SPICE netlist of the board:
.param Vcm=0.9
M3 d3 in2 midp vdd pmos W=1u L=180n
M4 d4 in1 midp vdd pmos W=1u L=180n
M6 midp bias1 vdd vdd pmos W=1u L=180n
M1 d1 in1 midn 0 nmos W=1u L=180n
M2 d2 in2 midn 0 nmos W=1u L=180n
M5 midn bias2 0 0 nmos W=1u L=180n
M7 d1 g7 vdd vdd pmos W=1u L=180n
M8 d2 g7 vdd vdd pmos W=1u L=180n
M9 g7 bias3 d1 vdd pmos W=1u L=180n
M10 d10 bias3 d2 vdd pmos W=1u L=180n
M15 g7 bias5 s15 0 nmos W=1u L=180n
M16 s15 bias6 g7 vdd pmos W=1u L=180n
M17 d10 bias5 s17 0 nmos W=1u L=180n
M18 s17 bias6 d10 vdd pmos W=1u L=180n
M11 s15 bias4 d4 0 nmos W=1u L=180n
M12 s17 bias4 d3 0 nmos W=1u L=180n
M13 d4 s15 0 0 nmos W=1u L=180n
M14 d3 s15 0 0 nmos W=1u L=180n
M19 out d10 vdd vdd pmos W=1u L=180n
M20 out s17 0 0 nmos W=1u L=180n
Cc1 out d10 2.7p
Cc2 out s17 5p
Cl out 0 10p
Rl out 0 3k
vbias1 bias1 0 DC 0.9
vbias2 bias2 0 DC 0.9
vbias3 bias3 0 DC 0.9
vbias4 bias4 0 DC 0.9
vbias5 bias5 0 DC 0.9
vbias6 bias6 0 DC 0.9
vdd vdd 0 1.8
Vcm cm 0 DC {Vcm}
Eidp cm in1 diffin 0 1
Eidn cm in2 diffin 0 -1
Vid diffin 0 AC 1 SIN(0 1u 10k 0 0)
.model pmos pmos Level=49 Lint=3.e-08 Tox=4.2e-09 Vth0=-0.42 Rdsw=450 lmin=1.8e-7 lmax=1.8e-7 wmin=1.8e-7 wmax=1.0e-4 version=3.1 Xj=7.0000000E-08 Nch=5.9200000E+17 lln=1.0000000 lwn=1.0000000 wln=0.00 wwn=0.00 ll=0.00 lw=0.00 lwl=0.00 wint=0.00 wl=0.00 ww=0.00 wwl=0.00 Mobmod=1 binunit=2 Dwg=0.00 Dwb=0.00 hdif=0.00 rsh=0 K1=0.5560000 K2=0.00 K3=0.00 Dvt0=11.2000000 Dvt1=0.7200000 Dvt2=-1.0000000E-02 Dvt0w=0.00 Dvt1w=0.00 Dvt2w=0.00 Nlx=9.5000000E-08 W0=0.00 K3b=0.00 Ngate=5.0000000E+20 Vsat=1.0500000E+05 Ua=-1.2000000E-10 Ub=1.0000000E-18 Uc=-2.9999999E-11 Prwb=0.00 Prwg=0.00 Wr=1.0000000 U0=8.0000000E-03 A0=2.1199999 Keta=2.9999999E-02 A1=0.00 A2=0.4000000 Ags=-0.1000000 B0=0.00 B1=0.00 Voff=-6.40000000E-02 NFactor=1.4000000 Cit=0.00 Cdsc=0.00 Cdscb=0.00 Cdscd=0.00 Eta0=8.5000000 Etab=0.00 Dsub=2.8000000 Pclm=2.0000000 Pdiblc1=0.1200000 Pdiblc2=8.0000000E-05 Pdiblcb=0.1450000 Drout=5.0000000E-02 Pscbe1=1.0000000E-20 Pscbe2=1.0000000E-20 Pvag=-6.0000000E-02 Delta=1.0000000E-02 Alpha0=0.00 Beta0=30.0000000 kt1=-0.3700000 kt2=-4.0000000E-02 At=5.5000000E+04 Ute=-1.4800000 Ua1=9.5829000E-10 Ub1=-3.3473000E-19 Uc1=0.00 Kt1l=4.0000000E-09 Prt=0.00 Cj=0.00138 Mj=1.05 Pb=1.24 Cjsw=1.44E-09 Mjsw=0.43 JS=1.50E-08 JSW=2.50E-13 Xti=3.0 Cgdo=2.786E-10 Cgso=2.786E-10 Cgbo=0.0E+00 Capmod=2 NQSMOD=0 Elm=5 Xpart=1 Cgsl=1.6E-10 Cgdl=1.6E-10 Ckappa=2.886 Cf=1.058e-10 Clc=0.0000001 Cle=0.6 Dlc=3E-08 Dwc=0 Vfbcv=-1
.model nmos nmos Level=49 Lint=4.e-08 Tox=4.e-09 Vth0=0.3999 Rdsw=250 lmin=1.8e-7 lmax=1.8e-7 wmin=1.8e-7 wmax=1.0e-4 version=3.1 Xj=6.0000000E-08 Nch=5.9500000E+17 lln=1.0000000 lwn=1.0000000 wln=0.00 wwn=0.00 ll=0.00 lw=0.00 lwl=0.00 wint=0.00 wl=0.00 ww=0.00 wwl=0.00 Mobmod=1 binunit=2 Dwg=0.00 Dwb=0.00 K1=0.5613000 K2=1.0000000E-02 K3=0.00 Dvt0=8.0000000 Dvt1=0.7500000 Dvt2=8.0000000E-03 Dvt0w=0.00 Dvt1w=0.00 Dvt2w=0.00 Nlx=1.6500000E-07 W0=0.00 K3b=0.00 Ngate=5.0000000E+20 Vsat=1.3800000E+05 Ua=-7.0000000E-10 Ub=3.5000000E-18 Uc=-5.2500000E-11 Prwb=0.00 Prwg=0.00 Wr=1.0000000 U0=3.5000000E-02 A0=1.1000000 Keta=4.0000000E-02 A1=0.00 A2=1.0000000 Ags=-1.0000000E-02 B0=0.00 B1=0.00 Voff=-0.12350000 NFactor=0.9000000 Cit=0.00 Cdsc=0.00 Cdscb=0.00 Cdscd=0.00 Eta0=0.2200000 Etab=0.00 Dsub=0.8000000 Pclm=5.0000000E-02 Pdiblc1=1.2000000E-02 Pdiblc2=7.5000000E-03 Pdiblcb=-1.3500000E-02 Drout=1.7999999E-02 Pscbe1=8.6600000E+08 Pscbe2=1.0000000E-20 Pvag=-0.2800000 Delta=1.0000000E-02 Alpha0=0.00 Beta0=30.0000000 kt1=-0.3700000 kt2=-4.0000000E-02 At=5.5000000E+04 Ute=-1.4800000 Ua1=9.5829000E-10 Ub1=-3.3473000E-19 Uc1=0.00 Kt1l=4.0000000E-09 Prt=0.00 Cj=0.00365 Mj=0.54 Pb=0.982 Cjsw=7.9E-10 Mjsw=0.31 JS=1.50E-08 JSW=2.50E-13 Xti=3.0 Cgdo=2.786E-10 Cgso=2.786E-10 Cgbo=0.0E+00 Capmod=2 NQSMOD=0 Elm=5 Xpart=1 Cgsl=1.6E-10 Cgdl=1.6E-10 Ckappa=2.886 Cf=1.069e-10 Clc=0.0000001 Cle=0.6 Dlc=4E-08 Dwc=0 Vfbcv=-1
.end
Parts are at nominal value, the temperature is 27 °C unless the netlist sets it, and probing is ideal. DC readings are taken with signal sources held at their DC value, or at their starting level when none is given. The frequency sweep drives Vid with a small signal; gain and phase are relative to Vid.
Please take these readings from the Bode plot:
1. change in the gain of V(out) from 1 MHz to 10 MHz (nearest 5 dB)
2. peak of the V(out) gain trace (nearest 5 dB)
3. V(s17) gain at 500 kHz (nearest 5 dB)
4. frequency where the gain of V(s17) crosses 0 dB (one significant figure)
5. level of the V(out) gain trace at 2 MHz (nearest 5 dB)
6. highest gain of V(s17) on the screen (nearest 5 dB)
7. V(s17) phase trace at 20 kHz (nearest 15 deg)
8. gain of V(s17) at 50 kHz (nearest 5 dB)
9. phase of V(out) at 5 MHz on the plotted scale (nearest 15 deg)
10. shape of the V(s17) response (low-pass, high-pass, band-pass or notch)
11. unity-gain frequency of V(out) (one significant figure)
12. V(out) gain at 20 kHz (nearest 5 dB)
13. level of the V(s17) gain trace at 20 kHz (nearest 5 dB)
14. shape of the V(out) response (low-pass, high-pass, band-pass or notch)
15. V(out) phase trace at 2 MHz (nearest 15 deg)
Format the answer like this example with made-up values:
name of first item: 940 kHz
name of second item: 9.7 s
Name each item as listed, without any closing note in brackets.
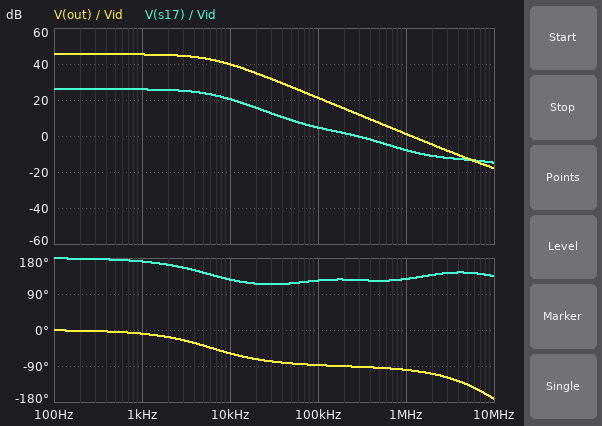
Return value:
change in the gain of V(out) from 1 MHz to 10 MHz: -20 dB
peak of the V(out) gain trace: 45 dB
V(s17) gain at 500 kHz: -5 dB
frequency where the gain of V(s17) crosses 0 dB: 300 kHz
level of the V(out) gain trace at 2 MHz: -5 dB
highest gain of V(s17) on the screen: 25 dB
V(s17) phase trace at 20 kHz: 120 deg
gain of V(s17) at 50 kHz: 10 dB
phase of V(out) at 5 MHz on the plotted scale: -135 deg
shape of the V(s17) response: low-pass
unity-gain frequency of V(out): 1 MHz
V(out) gain at 20 kHz: 35 dB
level of the V(s17) gain trace at 20 kHz: 15 dB
shape of the V(out) response: low-pass
V(out) phase trace at 2 MHz: -105 deg
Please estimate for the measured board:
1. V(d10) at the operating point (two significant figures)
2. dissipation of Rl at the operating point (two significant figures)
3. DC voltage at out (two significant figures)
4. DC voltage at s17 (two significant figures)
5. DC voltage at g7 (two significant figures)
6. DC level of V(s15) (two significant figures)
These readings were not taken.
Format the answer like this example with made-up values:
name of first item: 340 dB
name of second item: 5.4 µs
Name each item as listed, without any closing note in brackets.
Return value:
V(d10) at the operating point: 930 mV
dissipation of Rl at the operating point: 18 µW
DC voltage at out: 230 mV
DC voltage at s17: 550 mV
DC voltage at g7: 930 mV
DC level of V(s15): 550 mV
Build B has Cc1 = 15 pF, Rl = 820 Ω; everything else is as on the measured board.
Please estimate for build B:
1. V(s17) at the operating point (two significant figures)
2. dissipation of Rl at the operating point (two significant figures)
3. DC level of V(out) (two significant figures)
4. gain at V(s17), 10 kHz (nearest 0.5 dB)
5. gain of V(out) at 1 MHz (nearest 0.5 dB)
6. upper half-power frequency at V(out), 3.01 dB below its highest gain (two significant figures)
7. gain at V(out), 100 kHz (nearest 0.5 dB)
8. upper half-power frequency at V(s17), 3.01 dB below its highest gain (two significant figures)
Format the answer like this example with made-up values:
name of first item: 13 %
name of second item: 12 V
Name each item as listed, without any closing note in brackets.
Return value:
V(s17) at the operating point: 550 mV
dissipation of Rl at the operating point: 6.6 µW
DC level of V(out): 74 mV
gain at V(s17), 10 kHz: 17.5 dB
gain of V(out) at 1 MHz: -15.0 dB
upper half-power frequency at V(out), 3.01 dB below its highest gain: 2.3 kHz
gain at V(out), 100 kHz: 2.5 dB
upper half-power frequency at V(s17), 3.01 dB below its highest gain: 2.5 kHz
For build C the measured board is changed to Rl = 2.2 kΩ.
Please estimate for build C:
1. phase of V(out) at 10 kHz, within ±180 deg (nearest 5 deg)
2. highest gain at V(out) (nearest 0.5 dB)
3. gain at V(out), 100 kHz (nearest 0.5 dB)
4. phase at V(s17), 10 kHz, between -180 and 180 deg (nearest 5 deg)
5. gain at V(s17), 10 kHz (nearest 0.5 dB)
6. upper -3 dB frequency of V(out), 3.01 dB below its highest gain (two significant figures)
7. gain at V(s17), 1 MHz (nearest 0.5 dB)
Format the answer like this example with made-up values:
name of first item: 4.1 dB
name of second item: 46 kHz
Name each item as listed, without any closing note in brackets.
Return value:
phase of V(out) at 10 kHz, within ±180 deg: -55 deg
highest gain at V(out): 43.0 dB
gain at V(out), 100 kHz: 20.0 dB
phase at V(s17), 10 kHz, between -180 and 180 deg: 130 deg
gain at V(s17), 10 kHz: 21.5 dB
upper -3 dB frequency of V(out), 3.01 dB below its highest gain: 7.2 kHz
gain at V(s17), 1 MHz: -5.5 dB
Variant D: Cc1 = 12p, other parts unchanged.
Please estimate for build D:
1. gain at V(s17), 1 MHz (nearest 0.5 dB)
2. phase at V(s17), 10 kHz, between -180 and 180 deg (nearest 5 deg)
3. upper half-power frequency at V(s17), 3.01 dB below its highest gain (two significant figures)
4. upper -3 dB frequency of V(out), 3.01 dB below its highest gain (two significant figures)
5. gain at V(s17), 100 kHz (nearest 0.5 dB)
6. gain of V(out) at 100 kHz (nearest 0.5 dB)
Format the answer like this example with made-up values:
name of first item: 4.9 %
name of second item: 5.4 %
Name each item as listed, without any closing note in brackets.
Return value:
gain at V(s17), 1 MHz: -0.5 dB
phase at V(s17), 10 kHz, between -180 and 180 deg: 150 deg
upper half-power frequency at V(s17), 3.01 dB below its highest gain: 2.1 kHz
upper -3 dB frequency of V(out), 3.01 dB below its highest gain: 1.9 kHz
gain at V(s17), 100 kHz: 13.0 dB
gain of V(out) at 100 kHz: 12.5 dB
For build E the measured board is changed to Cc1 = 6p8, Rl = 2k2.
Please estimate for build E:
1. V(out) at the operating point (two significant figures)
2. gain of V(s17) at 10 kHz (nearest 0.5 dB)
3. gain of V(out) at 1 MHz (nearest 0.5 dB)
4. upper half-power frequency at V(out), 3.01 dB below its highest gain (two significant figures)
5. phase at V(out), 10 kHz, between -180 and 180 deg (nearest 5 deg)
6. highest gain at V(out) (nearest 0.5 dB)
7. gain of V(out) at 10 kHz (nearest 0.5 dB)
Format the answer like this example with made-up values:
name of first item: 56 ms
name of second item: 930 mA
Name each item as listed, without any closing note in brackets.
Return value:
V(out) at the operating point: 180 mV
gain of V(s17) at 10 kHz: 18.0 dB
gain of V(out) at 1 MHz: -4.5 dB
upper half-power frequency at V(out), 3.01 dB below its highest gain: 3.6 kHz
phase at V(out), 10 kHz, between -180 and 180 deg: -70 deg
highest gain at V(out): 43.0 dB
gain of V(out) at 10 kHz: 33.5 dB
